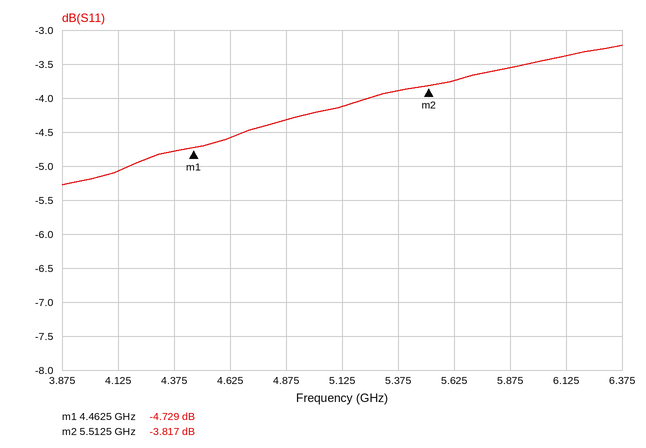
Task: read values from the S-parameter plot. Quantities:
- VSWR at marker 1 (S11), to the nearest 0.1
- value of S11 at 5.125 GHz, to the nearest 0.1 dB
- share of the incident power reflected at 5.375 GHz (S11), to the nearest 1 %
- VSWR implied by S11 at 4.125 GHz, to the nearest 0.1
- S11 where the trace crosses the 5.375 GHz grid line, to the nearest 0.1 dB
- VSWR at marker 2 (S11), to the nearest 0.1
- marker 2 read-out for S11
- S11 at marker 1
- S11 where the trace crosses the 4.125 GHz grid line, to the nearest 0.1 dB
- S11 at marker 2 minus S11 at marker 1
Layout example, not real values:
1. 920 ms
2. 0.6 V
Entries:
1. 3.8
2. -4.1 dB
3. 41 %
4. 3.5
5. -3.9 dB
6. 4.6
7. -3.817 dB
8. -4.729 dB
9. -5.1 dB
10. 0.912 dB
